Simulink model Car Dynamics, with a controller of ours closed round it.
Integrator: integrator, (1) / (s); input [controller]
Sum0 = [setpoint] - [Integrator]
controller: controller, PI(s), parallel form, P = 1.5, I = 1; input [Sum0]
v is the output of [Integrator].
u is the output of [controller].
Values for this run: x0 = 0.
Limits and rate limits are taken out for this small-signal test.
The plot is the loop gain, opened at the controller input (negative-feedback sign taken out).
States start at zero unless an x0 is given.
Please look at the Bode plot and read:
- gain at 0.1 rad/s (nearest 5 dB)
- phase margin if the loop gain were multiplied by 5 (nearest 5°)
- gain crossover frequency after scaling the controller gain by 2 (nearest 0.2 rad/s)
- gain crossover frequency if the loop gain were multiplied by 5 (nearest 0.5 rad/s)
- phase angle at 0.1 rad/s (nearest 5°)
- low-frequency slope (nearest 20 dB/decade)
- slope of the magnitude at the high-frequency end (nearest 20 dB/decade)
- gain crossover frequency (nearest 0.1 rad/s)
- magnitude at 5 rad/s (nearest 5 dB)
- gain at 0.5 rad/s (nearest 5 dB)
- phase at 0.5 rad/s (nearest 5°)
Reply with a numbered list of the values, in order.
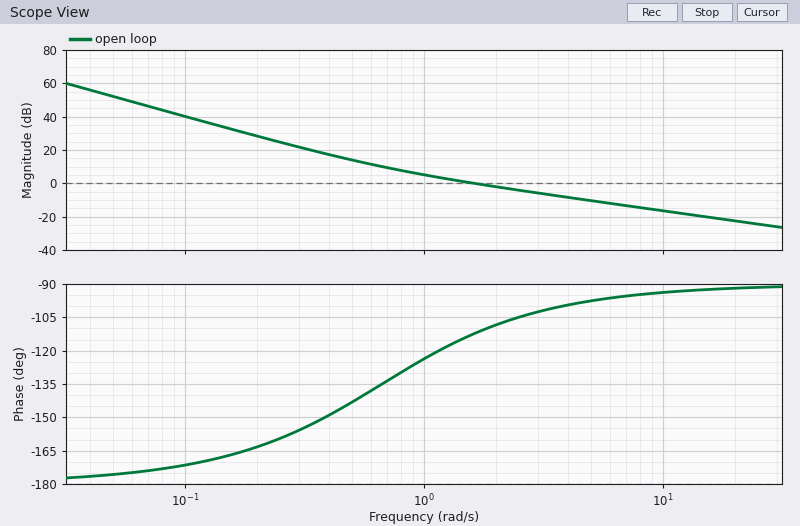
1. 40 dB
2. 85°
3. 3.0 rad/s
4. 7.5 rad/s
5. -170°
6. -40 dB/decade
7. -20 dB/decade
8. 1.6 rad/s
9. -10 dB
10. 15 dB
11. -145°
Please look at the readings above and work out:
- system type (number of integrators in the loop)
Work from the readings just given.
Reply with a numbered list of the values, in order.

1. 2
